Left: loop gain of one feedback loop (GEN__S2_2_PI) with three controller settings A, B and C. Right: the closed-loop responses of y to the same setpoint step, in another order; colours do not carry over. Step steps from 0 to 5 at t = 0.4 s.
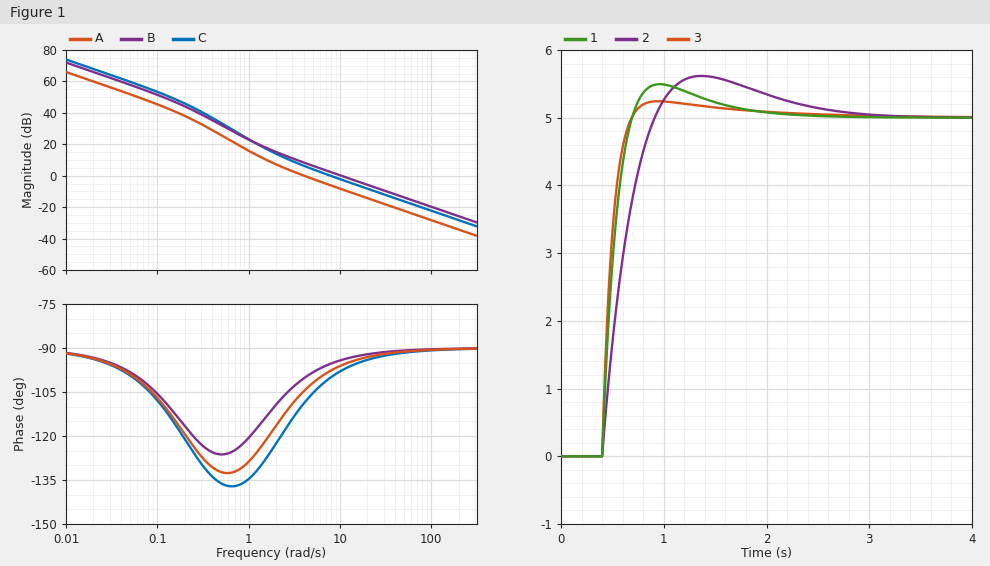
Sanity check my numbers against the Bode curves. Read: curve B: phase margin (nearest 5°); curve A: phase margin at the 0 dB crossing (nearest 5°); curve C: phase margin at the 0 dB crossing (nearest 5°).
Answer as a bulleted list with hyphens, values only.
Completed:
- 85°
- 75°
- 80°
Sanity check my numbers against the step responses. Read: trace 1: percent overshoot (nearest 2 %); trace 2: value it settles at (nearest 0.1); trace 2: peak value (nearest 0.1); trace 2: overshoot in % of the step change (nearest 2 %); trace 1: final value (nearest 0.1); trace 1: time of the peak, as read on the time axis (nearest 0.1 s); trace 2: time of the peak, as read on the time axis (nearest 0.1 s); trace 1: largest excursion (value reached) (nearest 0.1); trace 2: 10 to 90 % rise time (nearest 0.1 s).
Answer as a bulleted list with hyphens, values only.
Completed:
- 10 %
- 5.0
- 5.6
- 12 %
- 5.0
- 1.0 s
- 1.4 s
- 5.5
- 0.4 s
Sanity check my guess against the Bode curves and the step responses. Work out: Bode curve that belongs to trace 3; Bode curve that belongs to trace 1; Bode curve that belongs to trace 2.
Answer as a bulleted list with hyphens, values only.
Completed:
- B
- C
- A
